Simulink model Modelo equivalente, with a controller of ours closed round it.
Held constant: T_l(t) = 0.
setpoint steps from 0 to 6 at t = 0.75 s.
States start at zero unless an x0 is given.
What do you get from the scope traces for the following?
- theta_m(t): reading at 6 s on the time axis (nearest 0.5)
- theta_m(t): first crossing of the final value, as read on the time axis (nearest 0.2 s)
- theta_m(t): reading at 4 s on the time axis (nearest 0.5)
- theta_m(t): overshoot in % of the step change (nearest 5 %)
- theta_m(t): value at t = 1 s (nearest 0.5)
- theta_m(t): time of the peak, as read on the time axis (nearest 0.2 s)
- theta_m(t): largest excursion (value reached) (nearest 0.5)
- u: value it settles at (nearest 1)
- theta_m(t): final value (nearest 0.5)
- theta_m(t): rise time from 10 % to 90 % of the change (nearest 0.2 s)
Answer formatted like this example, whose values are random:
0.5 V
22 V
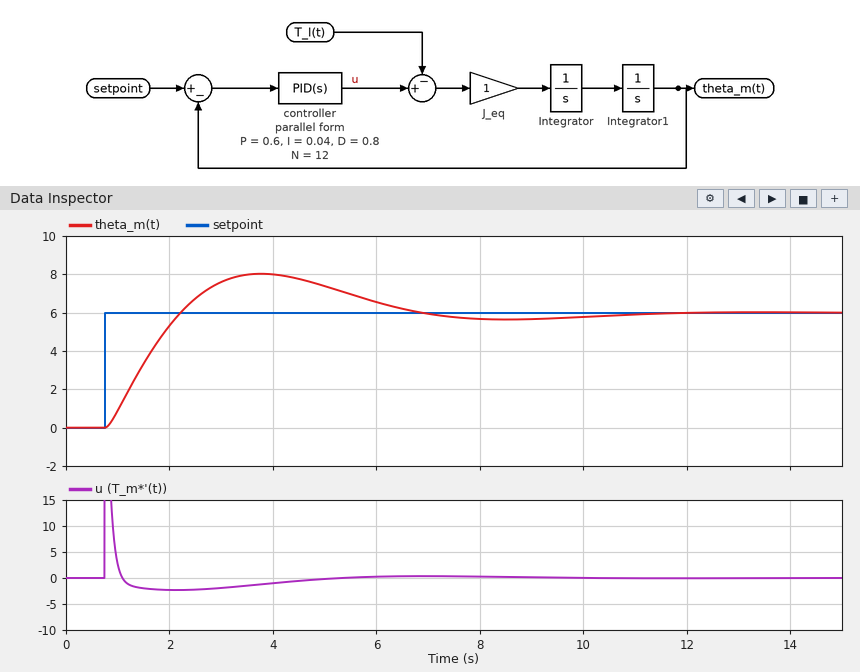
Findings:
6.5
2.2 s
8.0
35 %
1.0
3.8 s
8.0
0
6.0
1.0 s
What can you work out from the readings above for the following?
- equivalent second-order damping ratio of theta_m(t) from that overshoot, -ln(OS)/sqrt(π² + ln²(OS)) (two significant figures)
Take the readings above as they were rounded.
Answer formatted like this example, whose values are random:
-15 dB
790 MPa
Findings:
0.32
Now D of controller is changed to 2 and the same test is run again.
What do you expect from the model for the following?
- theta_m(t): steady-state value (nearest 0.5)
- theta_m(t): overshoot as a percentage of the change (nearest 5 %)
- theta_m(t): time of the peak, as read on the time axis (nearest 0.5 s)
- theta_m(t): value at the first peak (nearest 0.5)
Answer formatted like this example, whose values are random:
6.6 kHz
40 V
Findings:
6.0
10 %
3.0 s
6.5
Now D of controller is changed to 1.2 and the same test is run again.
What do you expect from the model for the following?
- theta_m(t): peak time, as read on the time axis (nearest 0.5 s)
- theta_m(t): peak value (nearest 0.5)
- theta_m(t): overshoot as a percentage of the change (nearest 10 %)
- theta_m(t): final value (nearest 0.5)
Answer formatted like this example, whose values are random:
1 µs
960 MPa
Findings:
3.5 s
7.5
20 %
6.0
